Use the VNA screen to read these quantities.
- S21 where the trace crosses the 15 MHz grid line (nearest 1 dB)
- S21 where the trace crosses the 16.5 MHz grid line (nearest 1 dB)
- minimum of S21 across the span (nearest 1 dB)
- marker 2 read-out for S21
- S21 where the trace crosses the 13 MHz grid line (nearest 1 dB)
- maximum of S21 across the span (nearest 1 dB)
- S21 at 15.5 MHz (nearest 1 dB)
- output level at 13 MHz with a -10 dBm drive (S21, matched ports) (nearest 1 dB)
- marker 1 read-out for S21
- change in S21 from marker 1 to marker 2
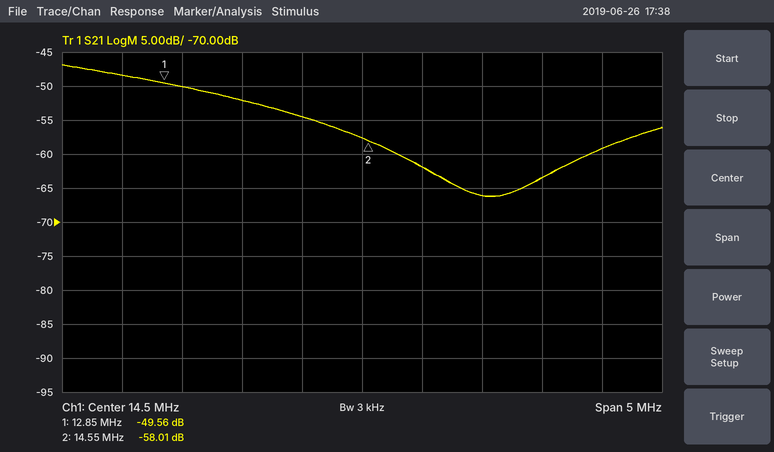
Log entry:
-62 dB
-59 dB
-66 dB
-58.01 dB
-50 dB
-47 dB
-66 dB
-60 dBm
-49.56 dB
-8.45 dB
